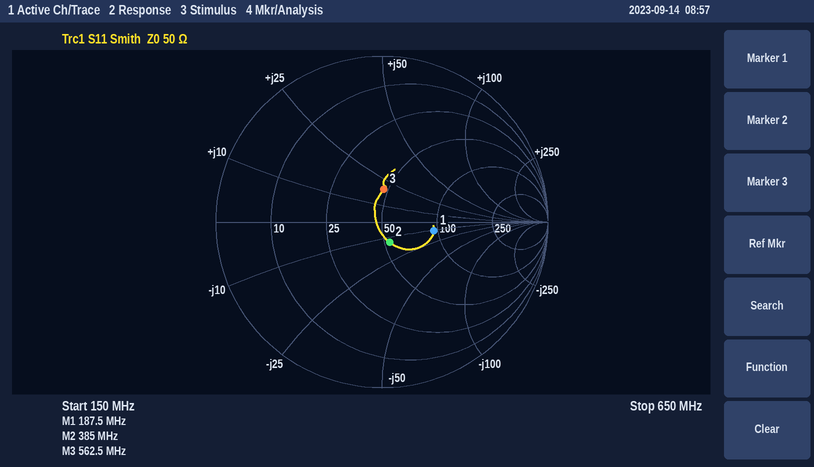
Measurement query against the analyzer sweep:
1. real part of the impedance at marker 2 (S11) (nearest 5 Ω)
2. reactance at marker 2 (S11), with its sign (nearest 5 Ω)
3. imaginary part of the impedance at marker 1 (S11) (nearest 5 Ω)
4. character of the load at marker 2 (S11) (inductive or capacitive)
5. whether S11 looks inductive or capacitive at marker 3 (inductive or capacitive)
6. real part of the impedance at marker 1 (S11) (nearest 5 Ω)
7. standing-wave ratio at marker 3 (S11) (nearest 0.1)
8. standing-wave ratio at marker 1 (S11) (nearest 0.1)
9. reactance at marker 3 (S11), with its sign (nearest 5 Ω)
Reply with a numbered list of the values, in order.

1. 55 Ω
2. -15 Ω
3. -10 Ω
4. capacitive
5. inductive
6. 95 Ω
7. 1.5
8. 1.9
9. +20 Ω
